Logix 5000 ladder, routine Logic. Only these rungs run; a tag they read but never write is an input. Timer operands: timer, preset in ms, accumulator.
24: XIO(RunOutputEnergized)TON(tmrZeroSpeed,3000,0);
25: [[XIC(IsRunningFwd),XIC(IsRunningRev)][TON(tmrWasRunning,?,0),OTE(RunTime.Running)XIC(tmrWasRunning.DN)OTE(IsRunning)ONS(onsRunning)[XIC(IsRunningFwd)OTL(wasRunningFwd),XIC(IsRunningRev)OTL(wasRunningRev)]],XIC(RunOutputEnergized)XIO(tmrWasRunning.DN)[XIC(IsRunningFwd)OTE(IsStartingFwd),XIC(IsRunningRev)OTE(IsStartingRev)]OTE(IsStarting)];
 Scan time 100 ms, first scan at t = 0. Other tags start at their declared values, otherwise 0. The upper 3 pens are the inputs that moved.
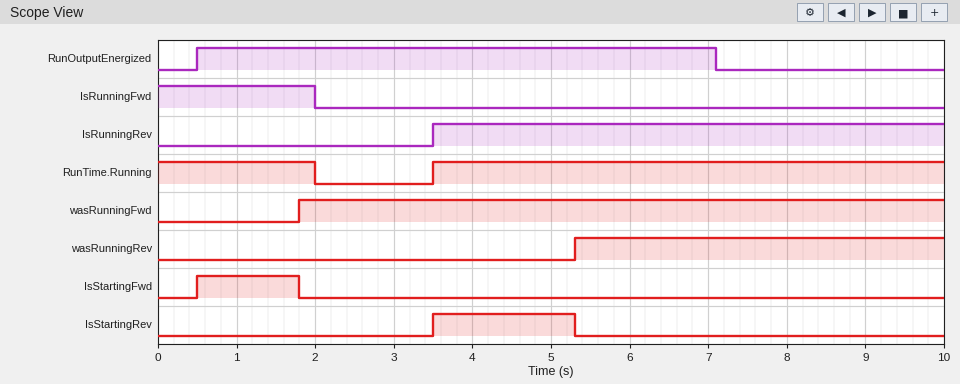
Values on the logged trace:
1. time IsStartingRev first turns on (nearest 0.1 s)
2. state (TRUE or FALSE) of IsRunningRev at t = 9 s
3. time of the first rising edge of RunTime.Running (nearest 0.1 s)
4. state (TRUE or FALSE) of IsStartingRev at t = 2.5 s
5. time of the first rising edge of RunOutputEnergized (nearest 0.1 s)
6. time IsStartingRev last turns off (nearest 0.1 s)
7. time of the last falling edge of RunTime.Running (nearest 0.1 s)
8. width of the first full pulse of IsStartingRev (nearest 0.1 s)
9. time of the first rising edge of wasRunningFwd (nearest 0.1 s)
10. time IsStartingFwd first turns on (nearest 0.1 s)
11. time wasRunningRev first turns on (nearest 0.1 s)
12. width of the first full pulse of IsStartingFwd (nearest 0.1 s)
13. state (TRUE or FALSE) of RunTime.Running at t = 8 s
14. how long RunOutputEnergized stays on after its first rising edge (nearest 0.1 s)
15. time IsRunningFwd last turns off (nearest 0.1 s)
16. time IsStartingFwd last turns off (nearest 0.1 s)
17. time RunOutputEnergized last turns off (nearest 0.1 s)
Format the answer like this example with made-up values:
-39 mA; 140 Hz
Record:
3.5 s; TRUE; 3.5 s; FALSE; 0.5 s; 5.3 s; 2.0 s; 1.8 s; 1.8 s; 0.5 s; 5.3 s; 1.3 s; TRUE; 6.6 s; 2.0 s; 1.8 s; 7.1 s
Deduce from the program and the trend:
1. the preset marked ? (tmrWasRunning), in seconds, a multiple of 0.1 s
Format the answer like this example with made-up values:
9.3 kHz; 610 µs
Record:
1.8 s
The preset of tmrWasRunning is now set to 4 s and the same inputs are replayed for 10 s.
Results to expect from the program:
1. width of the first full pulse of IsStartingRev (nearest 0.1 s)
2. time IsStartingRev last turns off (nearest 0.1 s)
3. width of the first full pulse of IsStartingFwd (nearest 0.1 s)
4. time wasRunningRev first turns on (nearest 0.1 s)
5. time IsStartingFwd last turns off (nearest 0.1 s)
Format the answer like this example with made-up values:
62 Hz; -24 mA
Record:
3.6 s; 7.1 s; 1.5 s; 7.5 s; 2.0 s
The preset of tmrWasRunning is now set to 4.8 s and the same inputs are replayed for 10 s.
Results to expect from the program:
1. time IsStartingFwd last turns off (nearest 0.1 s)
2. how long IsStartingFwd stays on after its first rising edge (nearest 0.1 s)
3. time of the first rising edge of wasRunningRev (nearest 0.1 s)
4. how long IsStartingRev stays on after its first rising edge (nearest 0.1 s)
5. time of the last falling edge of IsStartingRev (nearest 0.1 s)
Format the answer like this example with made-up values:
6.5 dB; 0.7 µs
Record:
2.0 s; 1.5 s; 8.3 s; 3.6 s; 7.1 s
